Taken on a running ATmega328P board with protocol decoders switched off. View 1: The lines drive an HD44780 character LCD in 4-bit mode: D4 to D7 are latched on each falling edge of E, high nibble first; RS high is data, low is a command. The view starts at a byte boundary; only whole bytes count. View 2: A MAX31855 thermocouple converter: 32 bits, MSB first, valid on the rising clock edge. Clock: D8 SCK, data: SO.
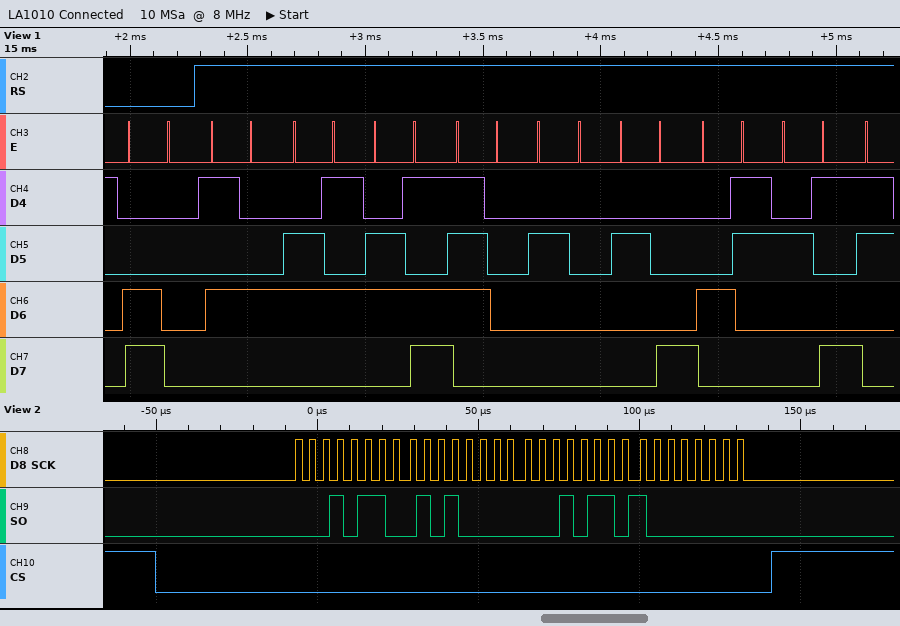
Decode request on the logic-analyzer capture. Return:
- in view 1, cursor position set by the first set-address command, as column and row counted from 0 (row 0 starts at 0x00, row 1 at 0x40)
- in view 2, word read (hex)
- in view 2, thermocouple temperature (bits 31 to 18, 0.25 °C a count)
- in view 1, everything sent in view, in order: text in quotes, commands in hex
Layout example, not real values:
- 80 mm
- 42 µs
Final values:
- column 0, row 1
- 0x16501680
- 357.00 °C
- 0xC0 "Temp (C)"
